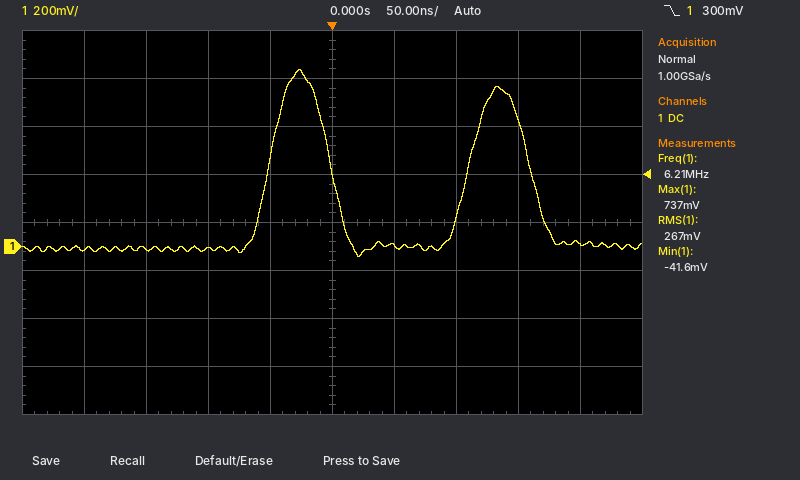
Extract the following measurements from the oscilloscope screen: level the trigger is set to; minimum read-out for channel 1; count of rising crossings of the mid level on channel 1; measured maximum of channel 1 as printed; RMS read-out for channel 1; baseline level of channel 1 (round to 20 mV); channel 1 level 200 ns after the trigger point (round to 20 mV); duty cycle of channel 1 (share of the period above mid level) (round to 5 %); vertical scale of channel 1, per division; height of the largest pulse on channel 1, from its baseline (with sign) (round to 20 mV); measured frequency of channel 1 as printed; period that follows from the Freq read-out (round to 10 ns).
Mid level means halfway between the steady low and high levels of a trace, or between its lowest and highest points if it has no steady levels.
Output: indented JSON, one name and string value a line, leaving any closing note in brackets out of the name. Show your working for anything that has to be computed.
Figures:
{
  "level the trigger is set to": "300 mV",
  "minimum read-out for channel 1": "-41.6 mV",
  "count of rising crossings of the mid level on channel 1": "2",
  "measured maximum of channel 1 as printed": "737 mV",
  "RMS read-out for channel 1": "267 mV",
  "baseline level of channel 1": "0 mV",
  "channel 1 level 200 ns after the trigger point": "20 mV",
  "duty cycle of channel 1 (share of the period above mid level)": "30 %",
  "vertical scale of channel 1, per division": "200 mV",
  "height of the largest pulse on channel 1, from its baseline (with sign)": "+740 mV",
  "measured frequency of channel 1 as printed": "6.21 MHz",
  "period that follows from the Freq read-out": "1 / 6.21 MHz ≈ 161 ns, so 160 ns to the nearest 10 ns"
}
